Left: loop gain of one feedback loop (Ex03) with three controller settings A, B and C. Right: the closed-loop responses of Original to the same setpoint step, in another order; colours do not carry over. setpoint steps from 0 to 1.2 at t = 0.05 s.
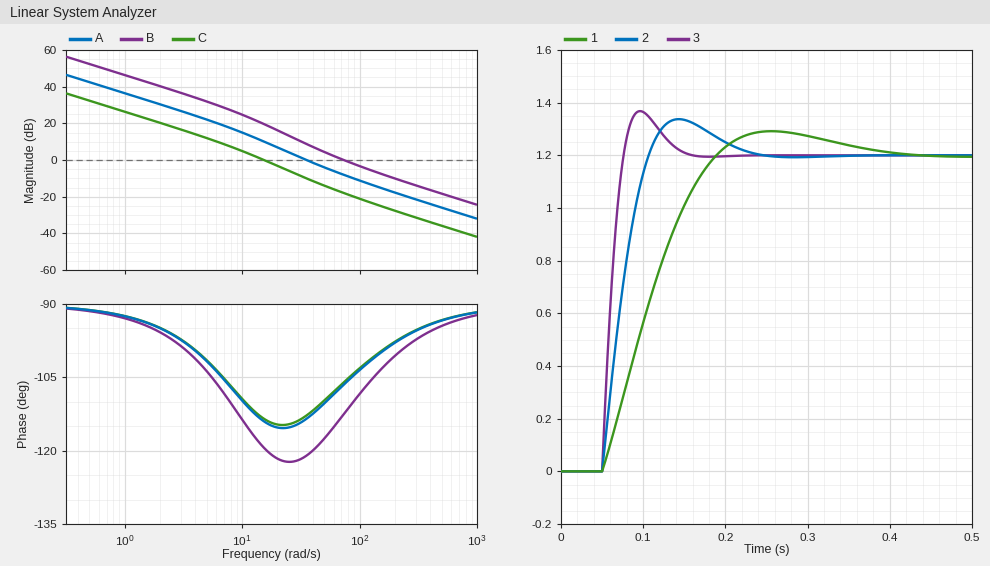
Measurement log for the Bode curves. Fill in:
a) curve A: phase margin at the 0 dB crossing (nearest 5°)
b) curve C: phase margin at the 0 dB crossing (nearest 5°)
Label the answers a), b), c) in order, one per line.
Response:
a) 65°
b) 65°
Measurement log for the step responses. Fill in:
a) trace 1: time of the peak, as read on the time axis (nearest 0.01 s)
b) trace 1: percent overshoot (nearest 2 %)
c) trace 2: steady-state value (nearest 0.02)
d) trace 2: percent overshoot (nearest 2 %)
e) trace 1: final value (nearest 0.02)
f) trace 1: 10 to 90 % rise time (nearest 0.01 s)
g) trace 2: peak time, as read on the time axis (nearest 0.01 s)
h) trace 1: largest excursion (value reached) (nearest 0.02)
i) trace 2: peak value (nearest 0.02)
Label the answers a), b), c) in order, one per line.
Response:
a) 0.26 s
b) 8 %
c) 1.20
d) 12 %
e) 1.20
f) 0.10 s
g) 0.14 s
h) 1.30
i) 1.34
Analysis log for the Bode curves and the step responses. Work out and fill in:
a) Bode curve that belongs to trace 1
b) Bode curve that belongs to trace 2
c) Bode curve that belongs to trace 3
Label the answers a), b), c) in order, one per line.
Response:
a) C
b) A
c) B
